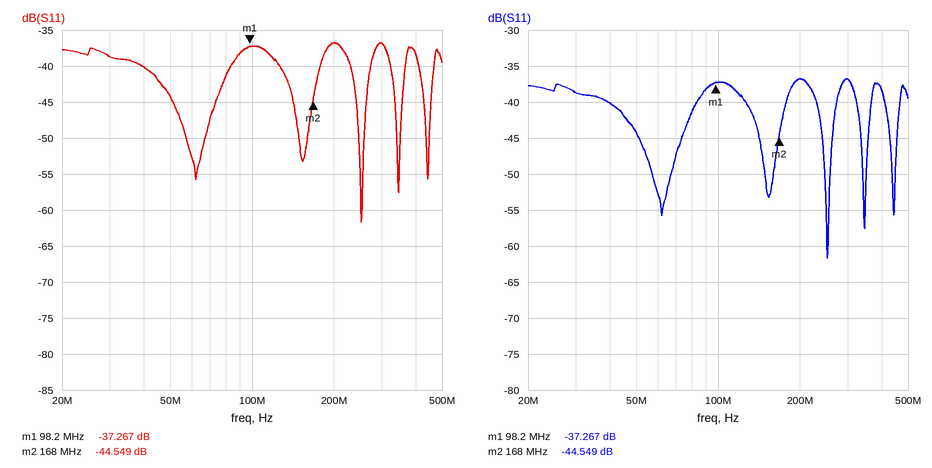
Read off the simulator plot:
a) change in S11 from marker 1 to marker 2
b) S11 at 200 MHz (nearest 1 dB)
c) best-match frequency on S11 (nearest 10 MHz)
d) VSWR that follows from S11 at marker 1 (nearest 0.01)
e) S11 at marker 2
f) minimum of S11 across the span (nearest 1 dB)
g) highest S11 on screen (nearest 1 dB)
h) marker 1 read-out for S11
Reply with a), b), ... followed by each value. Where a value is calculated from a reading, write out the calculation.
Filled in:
a) -44.549 − (-37.267) = -7.282 dB
b) -37 dB
c) 250 MHz
d) (1 + 0.0137)/(1 − 0.0137) ≈ 1.03
e) -44.549 dB
f) -62 dB
g) -37 dB
h) -37.267 dB
